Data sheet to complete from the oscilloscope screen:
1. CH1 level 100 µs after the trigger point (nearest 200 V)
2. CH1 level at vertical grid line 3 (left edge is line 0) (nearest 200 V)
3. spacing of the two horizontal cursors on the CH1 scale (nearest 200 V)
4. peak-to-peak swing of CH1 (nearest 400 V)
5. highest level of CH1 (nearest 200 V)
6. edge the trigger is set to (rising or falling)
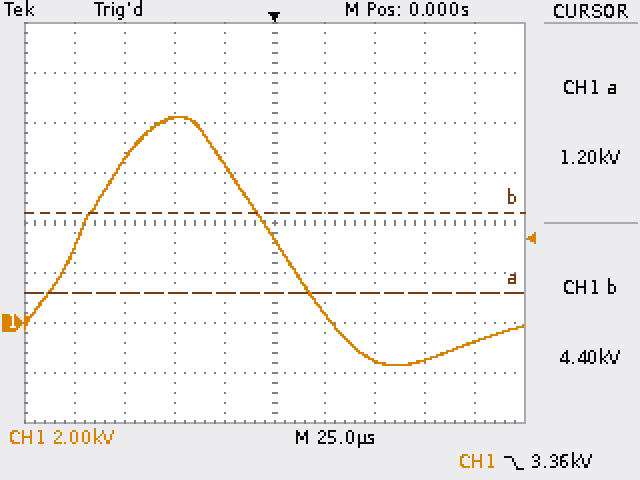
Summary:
-800 V
8.2 kV
3.2 kV
10.0 kV
8.2 kV
falling
